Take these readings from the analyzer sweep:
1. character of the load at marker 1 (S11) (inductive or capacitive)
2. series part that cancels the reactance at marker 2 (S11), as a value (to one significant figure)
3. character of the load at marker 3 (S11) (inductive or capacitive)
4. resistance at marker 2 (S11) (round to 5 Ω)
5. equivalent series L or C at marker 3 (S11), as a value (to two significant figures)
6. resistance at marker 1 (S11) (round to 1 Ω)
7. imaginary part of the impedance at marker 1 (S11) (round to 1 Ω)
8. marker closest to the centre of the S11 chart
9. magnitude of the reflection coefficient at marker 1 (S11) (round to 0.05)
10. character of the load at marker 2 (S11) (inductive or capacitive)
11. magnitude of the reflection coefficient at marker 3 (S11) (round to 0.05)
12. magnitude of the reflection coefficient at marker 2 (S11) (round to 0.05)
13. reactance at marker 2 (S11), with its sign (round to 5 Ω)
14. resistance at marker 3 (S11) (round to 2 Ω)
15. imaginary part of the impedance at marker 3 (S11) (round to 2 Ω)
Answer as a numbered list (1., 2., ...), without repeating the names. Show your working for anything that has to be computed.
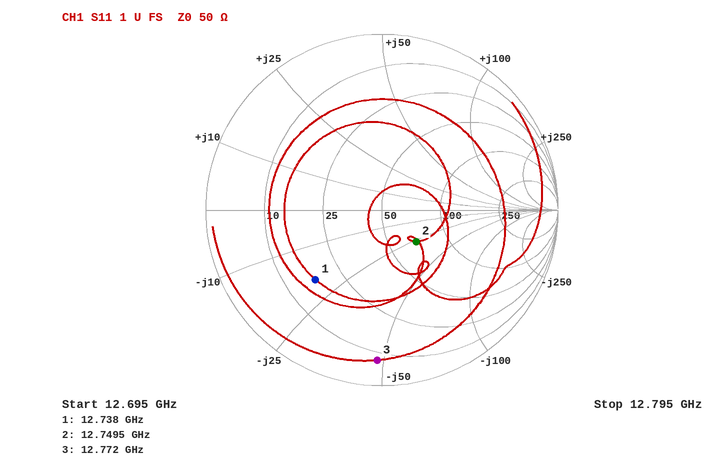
1. capacitive
2. L = 25 Ω/(2π × 12.7495 GHz) ≈ 312 pH, so 300 pH to one significant figure
3. capacitive
4. 70 Ω
5. C = 1/(2π × 12.772 GHz × 48 Ω) ≈ 260 fF
6. 17 Ω
7. -19 Ω
8. marker 2
9. 0.55
10. capacitive
11. 0.85
12. 0.25
13. -25 Ω
14. 8 Ω
15. -48 Ω
